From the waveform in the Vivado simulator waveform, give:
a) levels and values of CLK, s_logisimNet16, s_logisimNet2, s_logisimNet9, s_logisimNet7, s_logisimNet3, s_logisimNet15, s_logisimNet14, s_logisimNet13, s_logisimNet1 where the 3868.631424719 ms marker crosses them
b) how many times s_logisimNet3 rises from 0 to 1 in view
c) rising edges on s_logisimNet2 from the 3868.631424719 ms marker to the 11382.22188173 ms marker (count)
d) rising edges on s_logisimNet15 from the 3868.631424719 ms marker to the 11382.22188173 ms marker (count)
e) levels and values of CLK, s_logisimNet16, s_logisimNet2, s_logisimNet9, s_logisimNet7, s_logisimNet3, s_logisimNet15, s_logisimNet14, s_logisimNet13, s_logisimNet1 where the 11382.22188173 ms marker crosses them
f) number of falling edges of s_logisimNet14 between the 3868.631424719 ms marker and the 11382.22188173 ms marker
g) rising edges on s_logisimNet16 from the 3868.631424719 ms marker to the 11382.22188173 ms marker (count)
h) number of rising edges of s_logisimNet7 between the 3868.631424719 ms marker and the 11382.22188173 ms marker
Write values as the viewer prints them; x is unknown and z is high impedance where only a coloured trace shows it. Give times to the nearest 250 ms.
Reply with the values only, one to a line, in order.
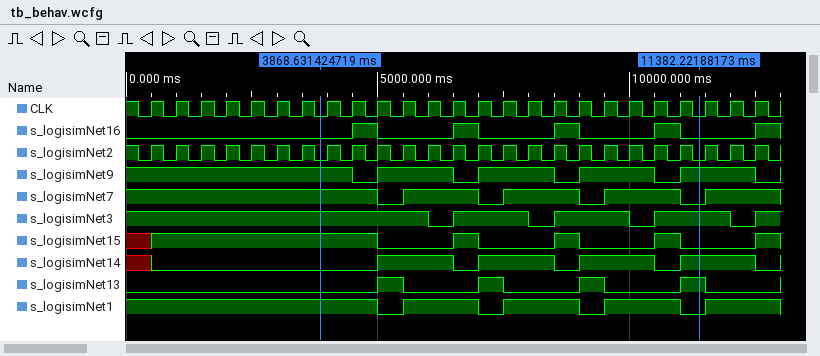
CLK=0, s_logisimNet16=0, s_logisimNet2=0, s_logisimNet9=1, s_logisimNet7=1, s_logisimNet3=1, s_logisimNet15=1, s_logisimNet14=0, s_logisimNet13=0, s_logisimNet1=1
4
15
3
CLK=0, s_logisimNet16=0, s_logisimNet2=0, s_logisimNet9=1, s_logisimNet7=0, s_logisimNet3=1, s_logisimNet15=0, s_logisimNet14=1, s_logisimNet13=1, s_logisimNet1=0
3
4
3
